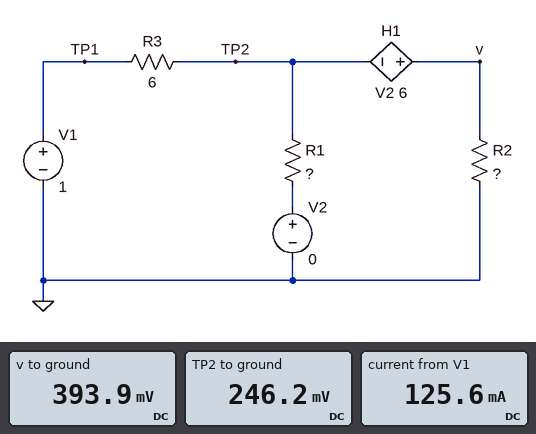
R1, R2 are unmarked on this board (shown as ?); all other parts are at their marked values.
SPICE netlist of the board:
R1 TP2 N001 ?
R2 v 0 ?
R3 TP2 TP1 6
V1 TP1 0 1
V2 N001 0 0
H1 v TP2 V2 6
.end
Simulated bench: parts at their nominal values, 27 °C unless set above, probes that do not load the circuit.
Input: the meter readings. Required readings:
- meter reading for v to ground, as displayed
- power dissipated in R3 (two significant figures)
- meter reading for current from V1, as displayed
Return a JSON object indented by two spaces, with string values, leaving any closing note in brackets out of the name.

{
  "meter reading for v to ground, as displayed": "393.9 mV",
  "power dissipated in R3": "95 mW",
  "meter reading for current from V1, as displayed": "125.6 mA"
}
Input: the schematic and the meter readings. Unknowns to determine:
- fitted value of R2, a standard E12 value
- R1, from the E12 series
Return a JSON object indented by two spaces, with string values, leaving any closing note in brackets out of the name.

{
  "fitted value of R2, a standard E12 value": "3.9 Ω",
  "R1, from the E12 series": "10 Ω"
}
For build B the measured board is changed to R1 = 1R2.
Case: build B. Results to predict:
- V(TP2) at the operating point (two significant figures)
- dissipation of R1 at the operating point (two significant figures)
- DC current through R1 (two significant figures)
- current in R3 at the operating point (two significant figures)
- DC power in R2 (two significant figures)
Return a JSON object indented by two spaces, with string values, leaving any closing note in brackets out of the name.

{
  "V(TP2) at the operating point": "66 mV",
  "dissipation of R1 at the operating point": "3.6 mW",
  "DC current through R1": "55 mA",
  "current in R3 at the operating point": "160 mA",
  "DC power in R2": "40 mW"
}
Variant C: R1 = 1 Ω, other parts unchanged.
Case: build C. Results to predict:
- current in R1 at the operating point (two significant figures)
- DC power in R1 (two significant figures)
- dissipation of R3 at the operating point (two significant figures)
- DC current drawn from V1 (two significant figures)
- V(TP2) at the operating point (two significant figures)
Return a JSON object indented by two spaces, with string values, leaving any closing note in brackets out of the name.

{
  "current in R1 at the operating point": "56 mA",
  "DC power in R1": "3.2 mW",
  "dissipation of R3 at the operating point": "150 mW",
  "DC current drawn from V1": "160 mA",
  "V(TP2) at the operating point": "56 mV"
}
